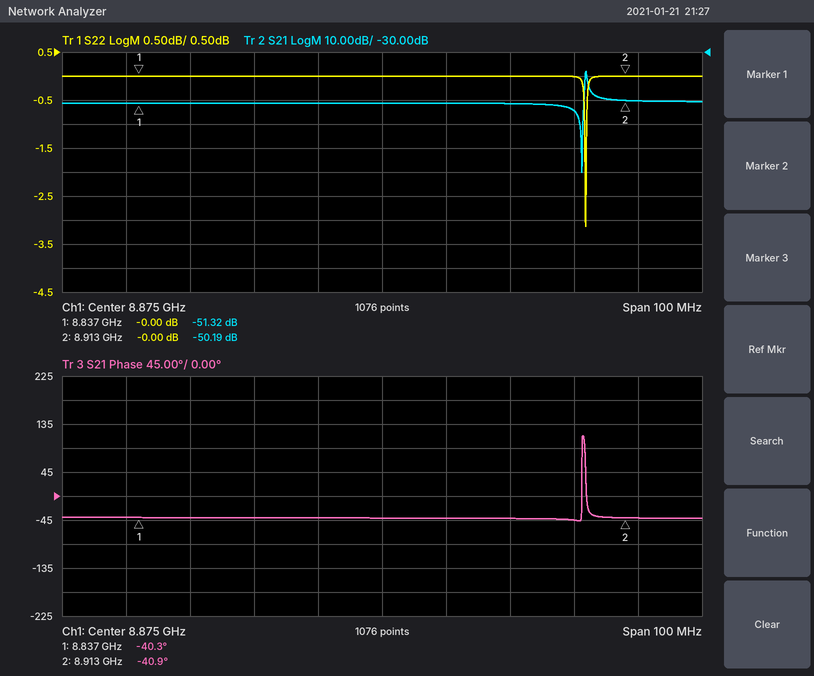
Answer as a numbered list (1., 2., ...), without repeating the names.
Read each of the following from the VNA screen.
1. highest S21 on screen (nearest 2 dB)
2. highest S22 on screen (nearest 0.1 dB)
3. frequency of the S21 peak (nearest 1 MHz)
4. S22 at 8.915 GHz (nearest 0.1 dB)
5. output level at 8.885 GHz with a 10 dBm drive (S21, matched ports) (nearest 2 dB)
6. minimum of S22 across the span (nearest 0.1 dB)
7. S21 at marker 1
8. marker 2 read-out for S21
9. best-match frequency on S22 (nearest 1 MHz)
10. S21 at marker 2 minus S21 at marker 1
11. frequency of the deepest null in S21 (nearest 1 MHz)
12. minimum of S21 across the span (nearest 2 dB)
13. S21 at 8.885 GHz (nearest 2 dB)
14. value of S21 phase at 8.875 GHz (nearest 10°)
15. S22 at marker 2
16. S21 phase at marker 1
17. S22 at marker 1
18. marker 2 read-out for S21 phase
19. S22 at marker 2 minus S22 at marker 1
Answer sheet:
1. -38 dB
2. 0.0 dB
3. 8.907 GHz
4. 0.0 dB
5. -42 dBm
6. -3.1 dB
7. -51.32 dB
8. -50.19 dB
9. 8.907 GHz
10. 1.13 dB
11. 8.906 GHz
12. -80 dB
13. -52 dB
14. -40°
15. -0.00 dB
16. -40.3°
17. -0.00 dB
18. -40.9°
19. 0.00 dB
